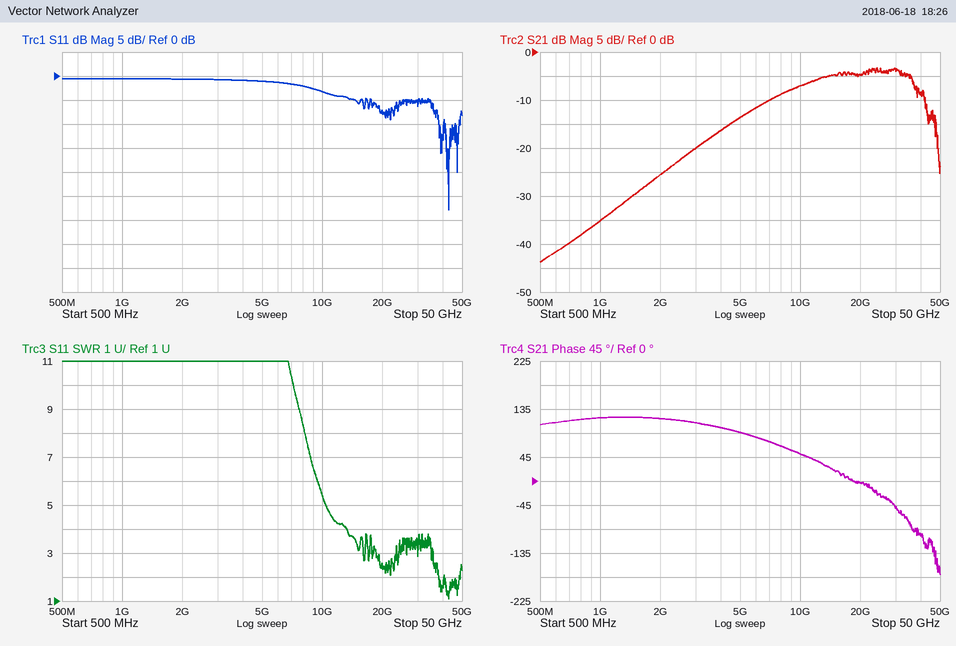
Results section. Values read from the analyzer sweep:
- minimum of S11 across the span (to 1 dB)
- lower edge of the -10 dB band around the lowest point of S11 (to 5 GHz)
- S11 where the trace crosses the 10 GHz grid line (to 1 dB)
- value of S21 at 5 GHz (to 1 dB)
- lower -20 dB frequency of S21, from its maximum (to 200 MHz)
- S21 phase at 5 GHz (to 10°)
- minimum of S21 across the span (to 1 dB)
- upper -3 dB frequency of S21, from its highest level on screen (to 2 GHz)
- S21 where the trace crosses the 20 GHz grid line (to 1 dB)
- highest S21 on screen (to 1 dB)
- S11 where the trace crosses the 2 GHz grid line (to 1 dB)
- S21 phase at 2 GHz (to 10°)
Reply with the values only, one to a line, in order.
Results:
-28 dB
40 GHz
-3 dB
-14 dB
2.4 GHz
90°
-44 dB
36 GHz
-5 dB
-3 dB
-1 dB
120°
